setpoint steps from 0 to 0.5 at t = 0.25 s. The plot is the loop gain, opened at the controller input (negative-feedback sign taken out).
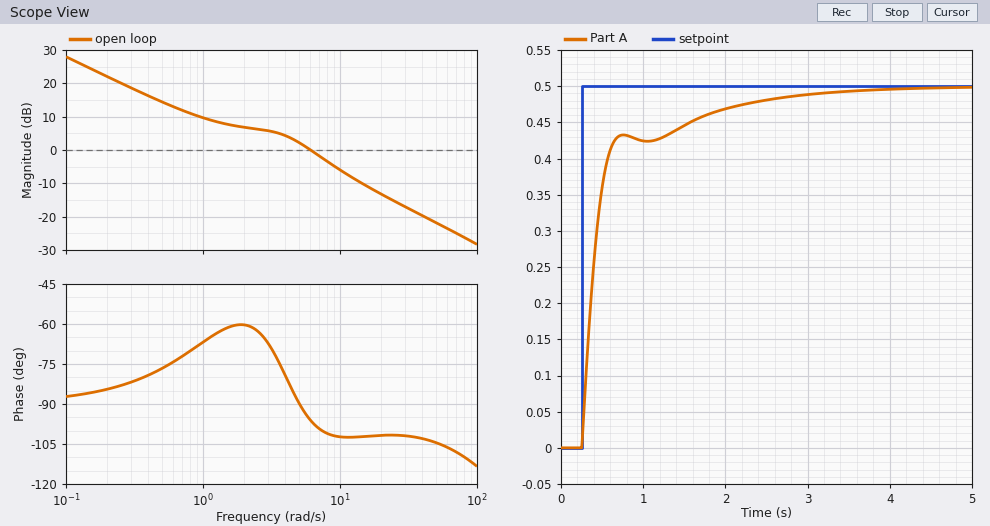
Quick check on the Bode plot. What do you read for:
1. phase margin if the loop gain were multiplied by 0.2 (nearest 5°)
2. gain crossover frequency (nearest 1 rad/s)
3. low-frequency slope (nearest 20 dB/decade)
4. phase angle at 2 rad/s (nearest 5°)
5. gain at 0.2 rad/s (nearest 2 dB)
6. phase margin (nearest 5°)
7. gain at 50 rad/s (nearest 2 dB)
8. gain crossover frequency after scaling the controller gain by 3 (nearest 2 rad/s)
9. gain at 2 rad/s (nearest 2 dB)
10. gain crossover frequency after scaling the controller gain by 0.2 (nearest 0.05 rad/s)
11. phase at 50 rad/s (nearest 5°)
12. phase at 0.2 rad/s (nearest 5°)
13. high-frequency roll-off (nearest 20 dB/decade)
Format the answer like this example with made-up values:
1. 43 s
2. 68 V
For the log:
1. 105°
2. 6 rad/s
3. -20 dB/decade
4. -60°
5. 22 dB
6. 85°
7. -22 dB
8. 14 rad/s
9. 6 dB
10. 0.55 rad/s
11. -105°
12. -85°
13. -20 dB/decade
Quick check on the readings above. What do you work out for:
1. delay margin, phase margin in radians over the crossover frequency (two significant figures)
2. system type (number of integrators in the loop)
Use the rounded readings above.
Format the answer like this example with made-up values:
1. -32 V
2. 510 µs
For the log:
1. 0.25 s
2. 1
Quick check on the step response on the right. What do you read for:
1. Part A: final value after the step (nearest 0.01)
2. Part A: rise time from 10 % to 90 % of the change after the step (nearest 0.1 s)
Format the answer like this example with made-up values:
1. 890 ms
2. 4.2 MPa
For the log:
1. 0.50
2. 1.3 s
